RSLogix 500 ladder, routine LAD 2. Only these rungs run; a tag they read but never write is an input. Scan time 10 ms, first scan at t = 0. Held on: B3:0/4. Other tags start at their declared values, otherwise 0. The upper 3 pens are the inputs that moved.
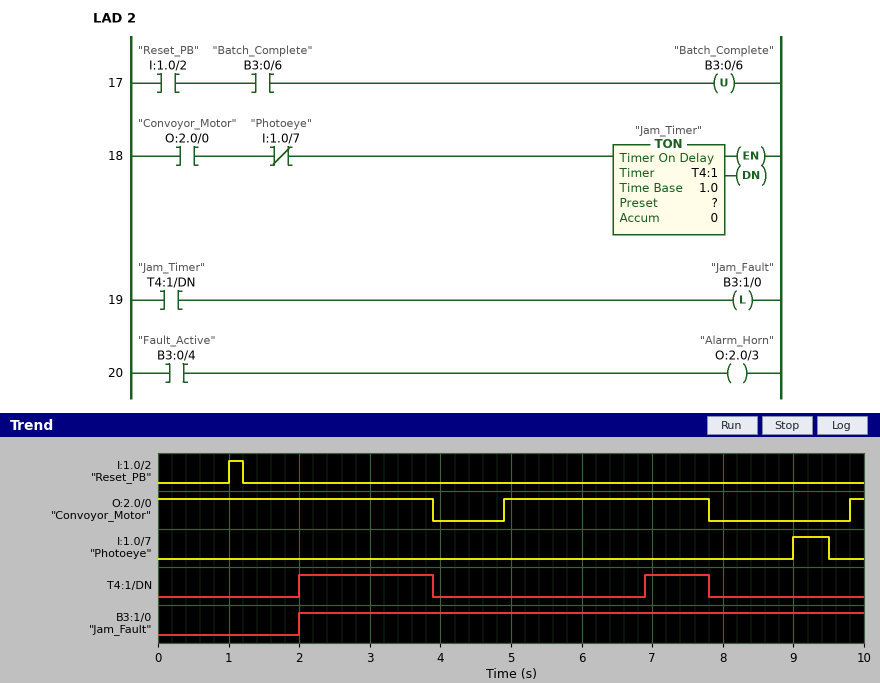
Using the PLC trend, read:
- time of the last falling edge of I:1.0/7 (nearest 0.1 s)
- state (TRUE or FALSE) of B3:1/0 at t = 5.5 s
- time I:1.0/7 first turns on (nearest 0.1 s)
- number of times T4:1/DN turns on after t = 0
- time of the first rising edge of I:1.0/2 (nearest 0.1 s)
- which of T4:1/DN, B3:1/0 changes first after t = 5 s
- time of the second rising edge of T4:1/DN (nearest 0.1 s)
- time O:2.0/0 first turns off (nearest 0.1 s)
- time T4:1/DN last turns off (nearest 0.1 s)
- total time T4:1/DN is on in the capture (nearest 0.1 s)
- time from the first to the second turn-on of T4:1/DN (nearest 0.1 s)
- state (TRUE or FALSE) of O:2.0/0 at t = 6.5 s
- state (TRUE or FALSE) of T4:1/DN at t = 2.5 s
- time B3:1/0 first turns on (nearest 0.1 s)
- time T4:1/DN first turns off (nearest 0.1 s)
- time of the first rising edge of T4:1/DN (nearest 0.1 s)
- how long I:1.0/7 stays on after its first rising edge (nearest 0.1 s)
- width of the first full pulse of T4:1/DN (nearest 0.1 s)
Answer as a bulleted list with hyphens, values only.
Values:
- 9.5 s
- TRUE
- 9.0 s
- 2
- 1.0 s
- T4:1/DN
- 6.9 s
- 3.9 s
- 7.8 s
- 2.8 s
- 4.9 s
- TRUE
- TRUE
- 2.0 s
- 3.9 s
- 2.0 s
- 0.5 s
- 1.9 s
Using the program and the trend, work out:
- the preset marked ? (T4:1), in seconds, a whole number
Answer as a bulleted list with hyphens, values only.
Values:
- 2 s
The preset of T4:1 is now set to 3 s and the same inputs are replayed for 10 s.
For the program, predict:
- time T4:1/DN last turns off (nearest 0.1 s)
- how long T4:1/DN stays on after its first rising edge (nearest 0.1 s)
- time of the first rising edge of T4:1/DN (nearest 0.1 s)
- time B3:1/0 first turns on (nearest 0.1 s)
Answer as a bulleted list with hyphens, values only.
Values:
- 3.9 s
- 0.9 s
- 3.0 s
- 3.0 s
